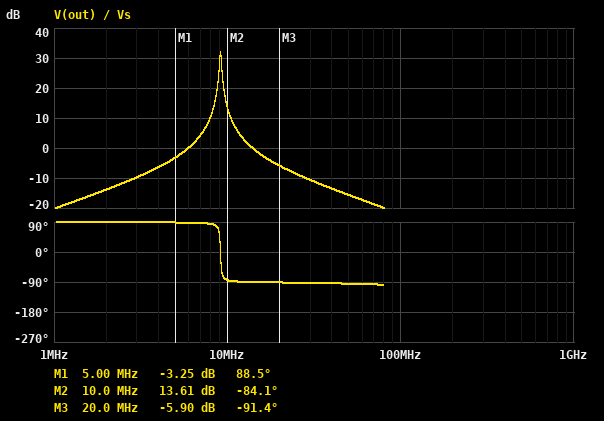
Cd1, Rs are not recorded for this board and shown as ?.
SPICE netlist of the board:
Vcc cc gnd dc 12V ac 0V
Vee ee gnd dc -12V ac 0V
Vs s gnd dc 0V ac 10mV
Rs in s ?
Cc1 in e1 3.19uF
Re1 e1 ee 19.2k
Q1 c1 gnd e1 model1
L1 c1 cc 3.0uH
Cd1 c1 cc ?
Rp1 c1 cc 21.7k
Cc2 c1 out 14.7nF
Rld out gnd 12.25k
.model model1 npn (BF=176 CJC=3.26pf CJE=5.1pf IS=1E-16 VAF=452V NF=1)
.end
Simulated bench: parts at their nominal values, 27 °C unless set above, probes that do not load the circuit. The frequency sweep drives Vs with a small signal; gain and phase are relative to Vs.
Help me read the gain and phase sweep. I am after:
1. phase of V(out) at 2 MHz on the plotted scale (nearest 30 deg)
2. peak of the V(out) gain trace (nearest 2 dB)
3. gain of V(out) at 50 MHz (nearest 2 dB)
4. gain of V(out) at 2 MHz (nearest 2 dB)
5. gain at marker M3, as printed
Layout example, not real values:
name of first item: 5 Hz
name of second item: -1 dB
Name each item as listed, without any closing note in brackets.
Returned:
phase of V(out) at 2 MHz on the plotted scale: 90 deg
peak of the V(out) gain trace: 32 dB
gain of V(out) at 50 MHz: -16 dB
gain of V(out) at 2 MHz: -14 dB
gain at marker M3, as printed: -5.90 dB
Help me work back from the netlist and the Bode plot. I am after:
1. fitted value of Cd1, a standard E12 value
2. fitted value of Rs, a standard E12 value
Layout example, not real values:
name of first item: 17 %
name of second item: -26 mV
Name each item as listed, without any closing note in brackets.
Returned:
fitted value of Cd1, a standard E12 value: 100 pF
fitted value of Rs, a standard E12 value: 150 Ω
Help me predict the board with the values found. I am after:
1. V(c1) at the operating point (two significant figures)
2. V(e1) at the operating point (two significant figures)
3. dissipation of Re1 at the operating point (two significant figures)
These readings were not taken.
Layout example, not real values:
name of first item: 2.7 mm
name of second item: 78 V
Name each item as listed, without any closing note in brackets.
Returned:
V(c1) at the operating point: 12 V
V(e1) at the operating point: -760 mV
dissipation of Re1 at the operating point: 6.6 mW
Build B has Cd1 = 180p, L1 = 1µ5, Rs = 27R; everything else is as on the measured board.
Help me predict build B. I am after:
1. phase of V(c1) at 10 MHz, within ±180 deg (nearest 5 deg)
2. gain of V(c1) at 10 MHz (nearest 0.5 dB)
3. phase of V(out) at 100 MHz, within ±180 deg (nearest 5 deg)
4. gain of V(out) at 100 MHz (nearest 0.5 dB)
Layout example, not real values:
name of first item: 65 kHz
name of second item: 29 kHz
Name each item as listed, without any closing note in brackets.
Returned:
phase of V(c1) at 10 MHz, within ±180 deg: -80 deg
gain of V(c1) at 10 MHz: 25.0 dB
phase of V(out) at 100 MHz, within ±180 deg: -95 deg
gain of V(out) at 100 MHz: -18.0 dB
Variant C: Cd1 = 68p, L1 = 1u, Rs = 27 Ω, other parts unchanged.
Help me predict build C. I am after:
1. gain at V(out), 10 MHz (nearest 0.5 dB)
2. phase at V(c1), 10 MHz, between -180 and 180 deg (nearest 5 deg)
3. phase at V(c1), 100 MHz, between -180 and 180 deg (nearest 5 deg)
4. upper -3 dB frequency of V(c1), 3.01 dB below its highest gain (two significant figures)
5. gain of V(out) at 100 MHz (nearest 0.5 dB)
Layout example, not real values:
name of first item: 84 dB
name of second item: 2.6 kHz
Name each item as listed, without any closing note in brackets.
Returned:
gain at V(out), 10 MHz: 1.5 dB
phase at V(c1), 10 MHz, between -180 and 180 deg: 90 deg
phase at V(c1), 100 MHz, between -180 and 180 deg: -95 deg
upper -3 dB frequency of V(c1), 3.01 dB below its highest gain: 19 MHz
gain of V(out) at 100 MHz: -9.5 dB
